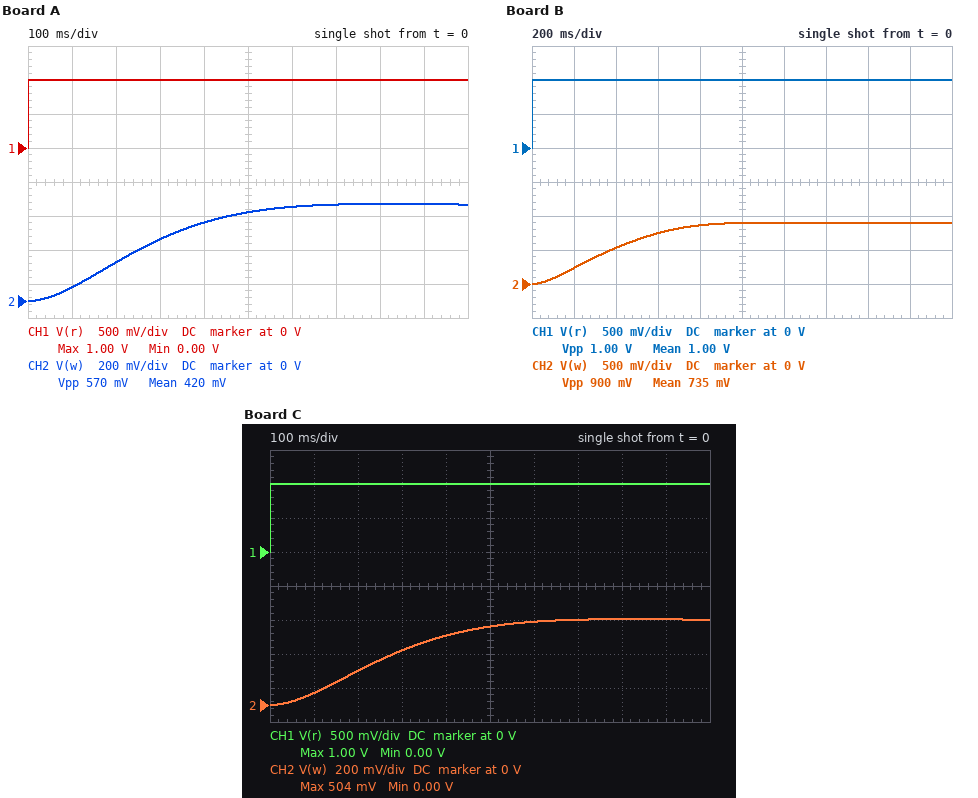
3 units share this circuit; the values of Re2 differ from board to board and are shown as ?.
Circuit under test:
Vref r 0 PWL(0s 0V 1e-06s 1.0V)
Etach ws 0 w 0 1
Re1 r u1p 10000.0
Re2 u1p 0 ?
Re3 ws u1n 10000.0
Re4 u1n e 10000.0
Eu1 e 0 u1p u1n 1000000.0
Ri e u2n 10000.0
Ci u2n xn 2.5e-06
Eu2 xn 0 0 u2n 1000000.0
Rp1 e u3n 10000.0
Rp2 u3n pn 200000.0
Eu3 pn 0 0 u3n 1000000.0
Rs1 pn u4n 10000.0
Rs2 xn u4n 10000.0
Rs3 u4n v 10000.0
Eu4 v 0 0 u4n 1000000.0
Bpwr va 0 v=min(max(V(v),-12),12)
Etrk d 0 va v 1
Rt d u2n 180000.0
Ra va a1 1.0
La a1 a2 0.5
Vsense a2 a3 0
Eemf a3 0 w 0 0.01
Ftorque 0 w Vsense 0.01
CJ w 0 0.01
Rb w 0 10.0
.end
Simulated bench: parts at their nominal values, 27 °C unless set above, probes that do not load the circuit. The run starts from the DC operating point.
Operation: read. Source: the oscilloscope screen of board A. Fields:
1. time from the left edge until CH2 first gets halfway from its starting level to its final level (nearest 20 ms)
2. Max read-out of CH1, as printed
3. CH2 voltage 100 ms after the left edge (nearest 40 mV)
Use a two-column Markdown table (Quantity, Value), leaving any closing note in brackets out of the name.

| Quantity | Value |
|---|---|
| time from the left edge until CH2 first gets halfway from its starting level to its final level | 240 ms |
| Max read-out of CH1, as printed | 1.00 V |
| CH2 voltage 100 ms after the left edge | 80 mV |
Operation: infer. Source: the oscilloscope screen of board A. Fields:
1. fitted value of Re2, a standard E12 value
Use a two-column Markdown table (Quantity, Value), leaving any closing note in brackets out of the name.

| Quantity | Value |
|---|---|
| fitted value of Re2, a standard E12 value | 3.9 kΩ |
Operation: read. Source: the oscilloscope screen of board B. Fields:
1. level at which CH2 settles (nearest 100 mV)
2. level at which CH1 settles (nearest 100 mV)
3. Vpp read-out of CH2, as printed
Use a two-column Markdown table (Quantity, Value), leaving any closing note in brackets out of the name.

| Quantity | Value |
|---|---|
| level at which CH2 settles | 900 mV |
| level at which CH1 settles | 1.0 V |
| Vpp read-out of CH2, as printed | 900 mV |
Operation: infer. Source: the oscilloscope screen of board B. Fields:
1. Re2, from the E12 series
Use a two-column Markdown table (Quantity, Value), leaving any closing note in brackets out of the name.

| Quantity | Value |
|---|---|
| Re2, from the E12 series | 8.2 kΩ |
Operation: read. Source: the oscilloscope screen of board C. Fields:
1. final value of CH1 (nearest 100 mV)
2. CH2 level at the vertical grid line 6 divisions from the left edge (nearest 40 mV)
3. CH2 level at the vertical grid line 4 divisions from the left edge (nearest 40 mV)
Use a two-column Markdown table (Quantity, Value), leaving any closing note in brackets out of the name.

| Quantity | Value |
|---|---|
| final value of CH1 | 1.0 V |
| CH2 level at the vertical grid line 6 divisions from the left edge | 480 mV |
| CH2 level at the vertical grid line 4 divisions from the left edge | 400 mV |
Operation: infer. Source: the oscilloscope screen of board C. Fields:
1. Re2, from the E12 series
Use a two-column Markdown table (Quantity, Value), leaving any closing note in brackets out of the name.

| Quantity | Value |
|---|---|
| Re2, from the E12 series | 3.3 kΩ |
